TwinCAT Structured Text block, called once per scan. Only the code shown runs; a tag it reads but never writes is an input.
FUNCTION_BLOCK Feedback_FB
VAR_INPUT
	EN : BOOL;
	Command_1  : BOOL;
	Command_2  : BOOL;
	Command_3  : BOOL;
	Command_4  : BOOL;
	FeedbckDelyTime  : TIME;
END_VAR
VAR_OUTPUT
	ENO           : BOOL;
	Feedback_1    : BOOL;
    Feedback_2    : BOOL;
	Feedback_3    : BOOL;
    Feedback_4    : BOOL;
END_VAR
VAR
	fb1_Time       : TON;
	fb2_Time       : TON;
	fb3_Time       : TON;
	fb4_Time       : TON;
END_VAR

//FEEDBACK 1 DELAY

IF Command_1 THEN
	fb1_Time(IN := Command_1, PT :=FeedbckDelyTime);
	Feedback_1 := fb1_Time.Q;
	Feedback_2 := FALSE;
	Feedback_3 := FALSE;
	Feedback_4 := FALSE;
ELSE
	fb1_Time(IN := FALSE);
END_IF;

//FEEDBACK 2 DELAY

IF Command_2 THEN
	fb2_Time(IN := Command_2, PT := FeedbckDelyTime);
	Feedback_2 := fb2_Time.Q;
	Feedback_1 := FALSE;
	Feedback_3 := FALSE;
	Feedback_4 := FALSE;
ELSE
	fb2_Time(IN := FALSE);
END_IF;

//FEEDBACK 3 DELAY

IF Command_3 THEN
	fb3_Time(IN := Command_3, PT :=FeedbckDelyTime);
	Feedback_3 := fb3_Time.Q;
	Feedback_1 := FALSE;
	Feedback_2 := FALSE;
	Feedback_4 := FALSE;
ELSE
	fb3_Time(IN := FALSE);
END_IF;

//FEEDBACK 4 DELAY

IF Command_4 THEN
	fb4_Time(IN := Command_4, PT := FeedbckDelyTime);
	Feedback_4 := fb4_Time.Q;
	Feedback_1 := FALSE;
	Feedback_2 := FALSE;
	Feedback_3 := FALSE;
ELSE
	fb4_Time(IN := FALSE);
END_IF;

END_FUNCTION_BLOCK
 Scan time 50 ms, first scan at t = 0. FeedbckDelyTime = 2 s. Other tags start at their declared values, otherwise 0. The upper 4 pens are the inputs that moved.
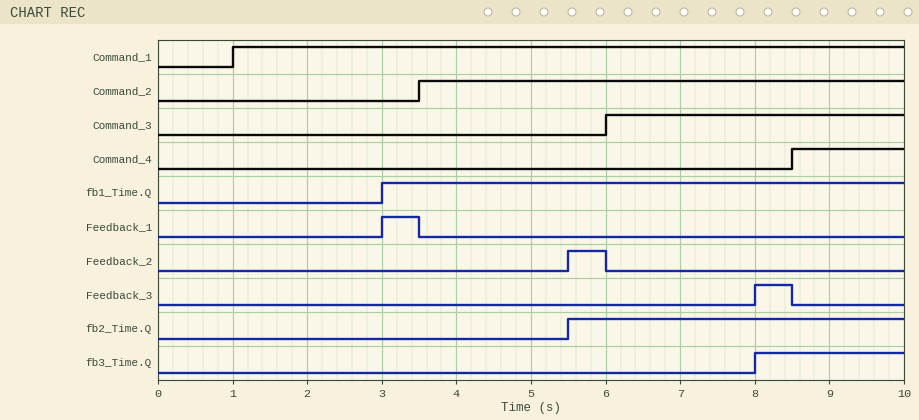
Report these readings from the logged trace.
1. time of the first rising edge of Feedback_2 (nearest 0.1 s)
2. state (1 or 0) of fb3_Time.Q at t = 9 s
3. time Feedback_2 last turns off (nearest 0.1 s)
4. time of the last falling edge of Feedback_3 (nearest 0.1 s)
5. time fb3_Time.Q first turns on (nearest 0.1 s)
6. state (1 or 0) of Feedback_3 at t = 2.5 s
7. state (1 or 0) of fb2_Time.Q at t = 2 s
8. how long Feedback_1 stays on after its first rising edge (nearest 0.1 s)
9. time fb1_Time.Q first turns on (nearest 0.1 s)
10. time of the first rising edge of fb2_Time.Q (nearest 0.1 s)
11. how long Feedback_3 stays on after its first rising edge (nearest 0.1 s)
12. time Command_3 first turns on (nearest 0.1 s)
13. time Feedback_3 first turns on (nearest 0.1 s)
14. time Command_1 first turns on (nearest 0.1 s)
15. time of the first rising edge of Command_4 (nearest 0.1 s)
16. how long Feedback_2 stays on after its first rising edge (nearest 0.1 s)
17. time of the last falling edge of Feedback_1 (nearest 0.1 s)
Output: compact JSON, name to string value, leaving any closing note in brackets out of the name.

{"time of the first rising edge of Feedback_2": "5.5 s", "state (1 or 0) of fb3_Time.Q at t = 9 s": "1", "time Feedback_2 last turns off": "6.0 s", "time of the last falling edge of Feedback_3": "8.5 s", "time fb3_Time.Q first turns on": "8.0 s", "state (1 or 0) of Feedback_3 at t = 2.5 s": "0", "state (1 or 0) of fb2_Time.Q at t = 2 s": "0", "how long Feedback_1 stays on after its first rising edge": "0.5 s", "time fb1_Time.Q first turns on": "3.0 s", "time of the first rising edge of fb2_Time.Q": "5.5 s", "how long Feedback_3 stays on after its first rising edge": "0.5 s", "time Command_3 first turns on": "6.0 s", "time Feedback_3 first turns on": "8.0 s", "time Command_1 first turns on": "1.0 s", "time of the first rising edge of Command_4": "8.5 s", "how long Feedback_2 stays on after its first rising edge": "0.5 s", "time of the last falling edge of Feedback_1": "3.5 s"}
